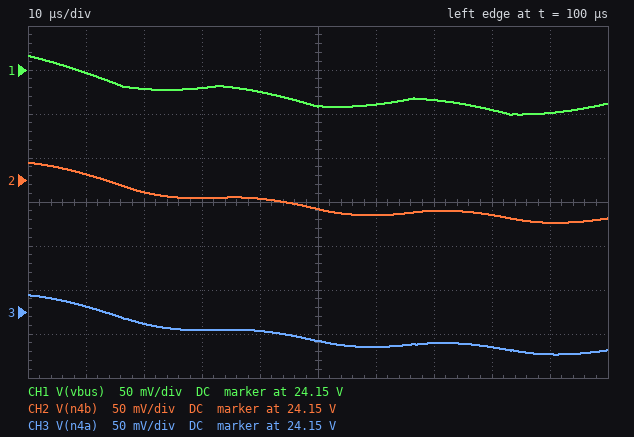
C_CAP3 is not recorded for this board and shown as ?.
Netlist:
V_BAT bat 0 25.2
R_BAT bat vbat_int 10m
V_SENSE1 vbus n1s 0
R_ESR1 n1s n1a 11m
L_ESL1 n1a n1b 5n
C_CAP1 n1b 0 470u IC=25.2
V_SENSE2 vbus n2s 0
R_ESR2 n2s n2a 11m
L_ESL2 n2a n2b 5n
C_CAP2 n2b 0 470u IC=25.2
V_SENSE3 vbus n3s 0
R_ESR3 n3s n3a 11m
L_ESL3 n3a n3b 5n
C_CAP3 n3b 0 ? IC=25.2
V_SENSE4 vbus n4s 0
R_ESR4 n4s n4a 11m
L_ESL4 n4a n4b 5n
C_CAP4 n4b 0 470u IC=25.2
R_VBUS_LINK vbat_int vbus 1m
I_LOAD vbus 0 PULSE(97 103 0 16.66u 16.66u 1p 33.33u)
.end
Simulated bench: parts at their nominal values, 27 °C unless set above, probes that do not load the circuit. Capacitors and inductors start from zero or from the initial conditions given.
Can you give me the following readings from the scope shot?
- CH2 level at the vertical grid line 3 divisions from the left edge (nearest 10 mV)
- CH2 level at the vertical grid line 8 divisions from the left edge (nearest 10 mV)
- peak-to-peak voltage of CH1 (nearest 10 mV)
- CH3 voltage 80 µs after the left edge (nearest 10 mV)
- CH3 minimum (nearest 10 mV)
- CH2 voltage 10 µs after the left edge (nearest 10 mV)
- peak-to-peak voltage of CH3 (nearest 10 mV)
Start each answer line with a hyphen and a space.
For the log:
- 24.13 V
- 24.11 V
- 70 mV
- 24.11 V
- 24.10 V
- 24.16 V
- 70 mV
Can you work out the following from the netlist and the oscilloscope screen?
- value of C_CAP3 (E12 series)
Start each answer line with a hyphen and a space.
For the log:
- 1.2 mF
